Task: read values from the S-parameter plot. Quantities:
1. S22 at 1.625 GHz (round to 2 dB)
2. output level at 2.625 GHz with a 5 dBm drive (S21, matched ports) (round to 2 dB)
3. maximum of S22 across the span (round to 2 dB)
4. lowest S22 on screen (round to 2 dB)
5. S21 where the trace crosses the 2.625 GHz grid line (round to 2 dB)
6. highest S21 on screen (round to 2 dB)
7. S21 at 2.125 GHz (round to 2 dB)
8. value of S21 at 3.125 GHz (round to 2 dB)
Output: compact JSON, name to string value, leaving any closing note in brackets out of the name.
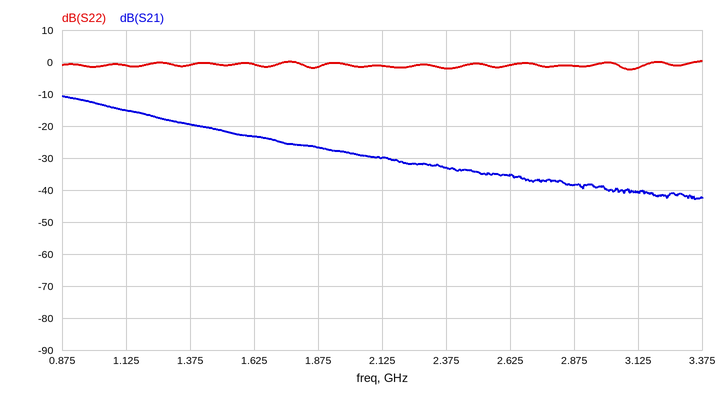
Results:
{"S22 at 1.625 GHz": "0 dB", "output level at 2.625 GHz with a 5 dBm drive (S21, matched ports)": "-30 dBm", "maximum of S22 across the span": "0 dB", "lowest S22 on screen": "-2 dB", "S21 where the trace crosses the 2.625 GHz grid line": "-36 dB", "highest S21 on screen": "-10 dB", "S21 at 2.125 GHz": "-30 dB", "value of S21 at 3.125 GHz": "-40 dB"}
